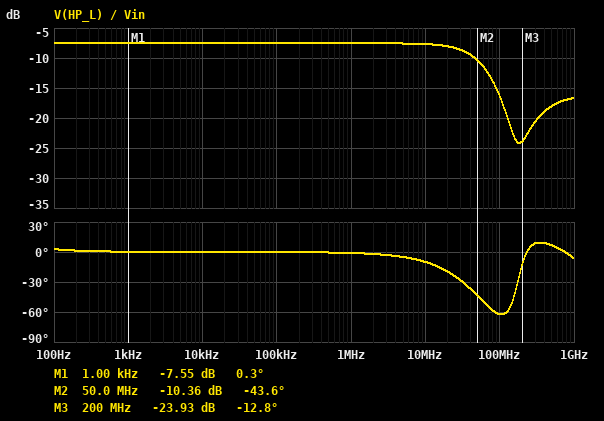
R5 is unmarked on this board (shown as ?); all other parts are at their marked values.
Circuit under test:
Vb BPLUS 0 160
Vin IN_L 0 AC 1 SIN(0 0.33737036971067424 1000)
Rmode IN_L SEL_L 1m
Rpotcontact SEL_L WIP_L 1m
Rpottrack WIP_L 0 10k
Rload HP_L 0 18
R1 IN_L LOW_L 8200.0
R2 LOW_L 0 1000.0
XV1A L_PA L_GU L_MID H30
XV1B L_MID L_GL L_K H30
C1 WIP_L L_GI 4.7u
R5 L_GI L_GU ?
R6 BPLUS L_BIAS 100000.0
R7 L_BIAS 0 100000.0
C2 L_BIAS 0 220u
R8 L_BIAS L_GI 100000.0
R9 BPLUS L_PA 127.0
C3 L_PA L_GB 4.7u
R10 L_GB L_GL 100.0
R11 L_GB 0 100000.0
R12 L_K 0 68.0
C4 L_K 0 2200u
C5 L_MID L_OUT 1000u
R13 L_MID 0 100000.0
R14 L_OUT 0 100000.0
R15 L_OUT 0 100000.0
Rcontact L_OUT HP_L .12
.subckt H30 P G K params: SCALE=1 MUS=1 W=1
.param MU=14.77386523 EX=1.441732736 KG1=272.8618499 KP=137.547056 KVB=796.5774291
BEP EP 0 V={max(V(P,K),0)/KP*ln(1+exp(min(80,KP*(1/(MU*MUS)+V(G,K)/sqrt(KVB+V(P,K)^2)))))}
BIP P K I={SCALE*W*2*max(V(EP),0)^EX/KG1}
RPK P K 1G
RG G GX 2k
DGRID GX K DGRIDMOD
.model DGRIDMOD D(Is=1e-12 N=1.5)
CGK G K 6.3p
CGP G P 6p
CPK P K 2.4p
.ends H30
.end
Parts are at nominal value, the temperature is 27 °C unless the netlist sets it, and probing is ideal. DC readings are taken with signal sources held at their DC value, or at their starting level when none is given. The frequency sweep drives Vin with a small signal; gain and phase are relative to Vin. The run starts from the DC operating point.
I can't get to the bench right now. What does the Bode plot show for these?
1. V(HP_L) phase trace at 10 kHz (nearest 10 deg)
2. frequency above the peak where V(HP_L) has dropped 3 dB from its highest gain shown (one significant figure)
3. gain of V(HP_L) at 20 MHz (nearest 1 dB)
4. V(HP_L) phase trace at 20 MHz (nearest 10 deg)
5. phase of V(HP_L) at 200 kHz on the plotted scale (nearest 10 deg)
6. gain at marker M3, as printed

0 deg
50 MHz
-8 dB
-20 deg
0 deg
-23.93 dB
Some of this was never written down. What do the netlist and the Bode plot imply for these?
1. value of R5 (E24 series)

56 Ω
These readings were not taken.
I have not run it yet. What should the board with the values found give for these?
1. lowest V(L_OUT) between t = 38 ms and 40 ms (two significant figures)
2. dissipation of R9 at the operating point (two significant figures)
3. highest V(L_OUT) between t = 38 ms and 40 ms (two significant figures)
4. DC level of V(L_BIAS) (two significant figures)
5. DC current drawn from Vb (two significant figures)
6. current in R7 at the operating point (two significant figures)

-140 mV
180 mW
140 mV
80 V
38 mA
800 µA
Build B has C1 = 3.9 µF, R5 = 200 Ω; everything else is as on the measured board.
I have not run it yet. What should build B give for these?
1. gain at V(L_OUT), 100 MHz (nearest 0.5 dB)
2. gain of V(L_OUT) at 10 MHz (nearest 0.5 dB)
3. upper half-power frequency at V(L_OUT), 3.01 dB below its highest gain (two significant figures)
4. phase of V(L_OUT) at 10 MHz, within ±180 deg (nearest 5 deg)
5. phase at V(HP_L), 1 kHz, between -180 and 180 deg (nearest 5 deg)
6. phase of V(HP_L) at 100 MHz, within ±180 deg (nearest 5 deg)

-22.0 dB
-8.0 dB
34 MHz
-20 deg
0 deg
-90 deg
